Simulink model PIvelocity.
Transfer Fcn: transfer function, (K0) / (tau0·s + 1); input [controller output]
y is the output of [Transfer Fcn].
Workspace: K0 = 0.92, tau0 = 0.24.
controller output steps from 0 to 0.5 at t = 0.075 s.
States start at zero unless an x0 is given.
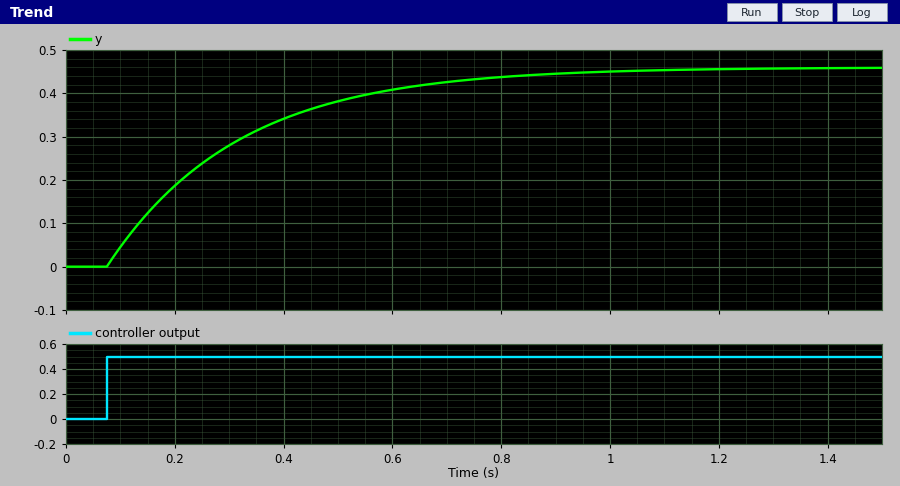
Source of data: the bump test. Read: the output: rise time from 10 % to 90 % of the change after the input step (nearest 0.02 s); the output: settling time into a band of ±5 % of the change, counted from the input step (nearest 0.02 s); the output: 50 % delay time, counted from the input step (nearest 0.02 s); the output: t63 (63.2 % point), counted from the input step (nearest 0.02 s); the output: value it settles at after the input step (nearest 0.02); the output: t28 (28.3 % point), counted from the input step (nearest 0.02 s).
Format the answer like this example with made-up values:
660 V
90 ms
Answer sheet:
0.52 s
0.72 s
0.16 s
0.24 s
0.46
0.08 s
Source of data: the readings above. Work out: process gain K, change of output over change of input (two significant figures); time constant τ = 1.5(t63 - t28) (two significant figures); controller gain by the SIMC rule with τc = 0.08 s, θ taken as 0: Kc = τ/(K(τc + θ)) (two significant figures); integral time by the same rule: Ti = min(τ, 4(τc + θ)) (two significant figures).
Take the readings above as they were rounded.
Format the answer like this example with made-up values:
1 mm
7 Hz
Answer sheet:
0.92
0.24 s
3.3
0.24 s
